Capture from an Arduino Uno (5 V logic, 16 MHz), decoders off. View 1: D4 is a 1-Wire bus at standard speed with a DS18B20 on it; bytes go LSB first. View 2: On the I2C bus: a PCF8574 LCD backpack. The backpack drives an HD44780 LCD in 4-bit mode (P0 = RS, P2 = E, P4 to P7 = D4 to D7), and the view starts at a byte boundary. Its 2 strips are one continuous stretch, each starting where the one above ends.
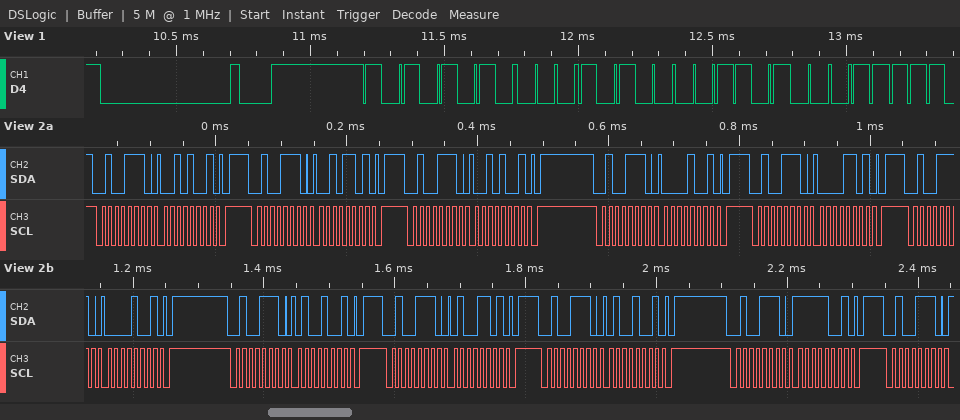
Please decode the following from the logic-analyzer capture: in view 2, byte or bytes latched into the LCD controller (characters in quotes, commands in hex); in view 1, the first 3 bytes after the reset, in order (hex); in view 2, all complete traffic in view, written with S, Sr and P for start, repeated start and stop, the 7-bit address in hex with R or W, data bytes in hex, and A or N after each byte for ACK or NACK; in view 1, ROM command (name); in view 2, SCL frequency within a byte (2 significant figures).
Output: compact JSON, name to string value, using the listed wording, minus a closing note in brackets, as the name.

{"in view 2, byte or bytes latched into the LCD controller": "' '", "in view 1, the first 3 bytes after the reset, in order": "55 28 2C", "in view 2, all complete traffic in view, written with S, Sr and P for start, repeated start and stop, the 7-bit address in hex with R or W, data bytes in hex, and A or N after each byte for ACK or NACK": "S 27W A 29 A P S 27W A 2D A P S 27W A 29 A P S 27W A 09 A P S 27W A 0D A P S 27W A 09 A P S 27W A 49 A P S 27W A 4D A P S 27W A 49 A P S 27W A F9 A P S 27W A", "in view 1, ROM command": "Match ROM", "in view 2, SCL frequency within a byte": "100 kHz"}
